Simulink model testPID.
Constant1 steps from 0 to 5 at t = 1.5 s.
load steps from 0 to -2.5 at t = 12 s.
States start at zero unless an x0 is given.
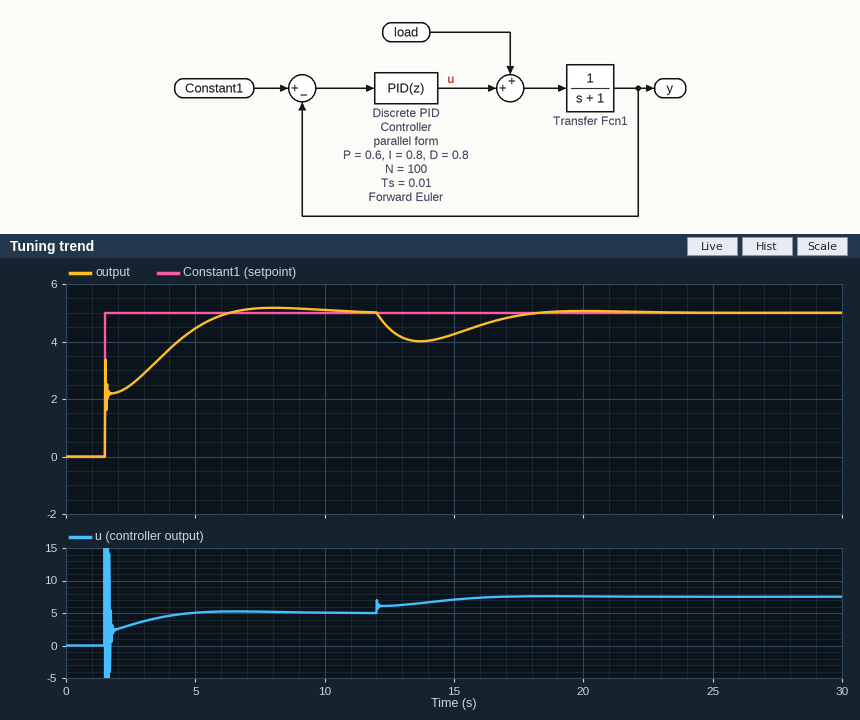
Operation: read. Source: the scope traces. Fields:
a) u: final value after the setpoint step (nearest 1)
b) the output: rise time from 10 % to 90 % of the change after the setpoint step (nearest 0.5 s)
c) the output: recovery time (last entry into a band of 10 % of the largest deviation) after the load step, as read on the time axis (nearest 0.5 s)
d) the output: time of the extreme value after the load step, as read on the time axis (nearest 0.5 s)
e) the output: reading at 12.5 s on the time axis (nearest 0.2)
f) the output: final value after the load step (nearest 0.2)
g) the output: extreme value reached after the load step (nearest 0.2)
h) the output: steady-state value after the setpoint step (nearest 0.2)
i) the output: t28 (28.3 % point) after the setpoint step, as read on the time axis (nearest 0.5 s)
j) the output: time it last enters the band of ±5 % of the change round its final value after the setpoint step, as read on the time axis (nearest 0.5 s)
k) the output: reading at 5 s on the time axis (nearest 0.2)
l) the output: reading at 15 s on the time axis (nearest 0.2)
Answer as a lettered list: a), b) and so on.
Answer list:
a) 5
b) 3.5 s
c) 17.5 s
d) 13.5 s
e) 4.4
f) 5.0
g) 4.0
h) 5.0
i) 1.5 s
j) 5.5 s
k) 4.4
l) 4.2
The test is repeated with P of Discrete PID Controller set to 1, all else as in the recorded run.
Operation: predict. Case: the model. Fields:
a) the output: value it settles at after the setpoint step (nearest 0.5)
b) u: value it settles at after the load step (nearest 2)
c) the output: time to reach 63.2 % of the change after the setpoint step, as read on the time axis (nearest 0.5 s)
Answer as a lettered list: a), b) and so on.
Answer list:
a) 5.0
b) 8
c) 1.5 s
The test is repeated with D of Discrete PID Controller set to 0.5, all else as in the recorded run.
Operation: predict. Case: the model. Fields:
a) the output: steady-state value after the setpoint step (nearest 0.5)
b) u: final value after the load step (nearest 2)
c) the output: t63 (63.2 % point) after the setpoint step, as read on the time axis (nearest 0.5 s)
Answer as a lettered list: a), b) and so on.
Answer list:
a) 5.0
b) 8
c) 3.0 s
